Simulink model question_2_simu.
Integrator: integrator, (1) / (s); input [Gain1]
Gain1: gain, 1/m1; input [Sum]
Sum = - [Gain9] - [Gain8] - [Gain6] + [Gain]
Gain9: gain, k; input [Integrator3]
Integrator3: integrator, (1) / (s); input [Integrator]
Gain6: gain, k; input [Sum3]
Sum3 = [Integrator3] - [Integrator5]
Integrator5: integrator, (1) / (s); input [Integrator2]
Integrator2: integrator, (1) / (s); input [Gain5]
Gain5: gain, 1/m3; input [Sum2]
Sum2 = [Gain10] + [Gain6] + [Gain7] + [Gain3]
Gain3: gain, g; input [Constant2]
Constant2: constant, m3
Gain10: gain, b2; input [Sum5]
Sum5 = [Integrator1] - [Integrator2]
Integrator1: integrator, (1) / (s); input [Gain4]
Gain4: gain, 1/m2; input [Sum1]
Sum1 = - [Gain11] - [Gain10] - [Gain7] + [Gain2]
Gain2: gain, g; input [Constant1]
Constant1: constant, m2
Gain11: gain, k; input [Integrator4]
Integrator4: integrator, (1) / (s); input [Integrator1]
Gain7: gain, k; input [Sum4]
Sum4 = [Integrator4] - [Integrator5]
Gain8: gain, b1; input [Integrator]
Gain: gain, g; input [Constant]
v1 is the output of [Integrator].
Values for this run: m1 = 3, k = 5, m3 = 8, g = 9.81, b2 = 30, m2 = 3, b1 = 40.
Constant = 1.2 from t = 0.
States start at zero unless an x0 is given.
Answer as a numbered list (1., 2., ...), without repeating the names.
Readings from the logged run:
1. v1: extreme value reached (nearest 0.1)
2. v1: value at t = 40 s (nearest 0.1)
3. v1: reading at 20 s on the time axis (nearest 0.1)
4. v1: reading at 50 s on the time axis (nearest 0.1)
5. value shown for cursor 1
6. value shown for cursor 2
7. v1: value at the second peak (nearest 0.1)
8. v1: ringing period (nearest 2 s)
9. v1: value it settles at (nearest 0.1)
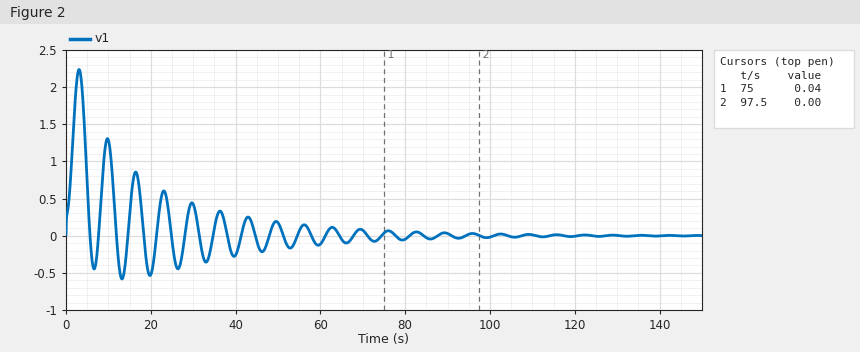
1. 2.2
2. -0.3
3. -0.5
4. 0.2
5. 0.04
6. 0.00
7. 1.3
8. 6 s
9. 0.0
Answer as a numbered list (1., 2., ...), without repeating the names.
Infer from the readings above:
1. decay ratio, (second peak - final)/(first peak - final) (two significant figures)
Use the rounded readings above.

1. 0.59
